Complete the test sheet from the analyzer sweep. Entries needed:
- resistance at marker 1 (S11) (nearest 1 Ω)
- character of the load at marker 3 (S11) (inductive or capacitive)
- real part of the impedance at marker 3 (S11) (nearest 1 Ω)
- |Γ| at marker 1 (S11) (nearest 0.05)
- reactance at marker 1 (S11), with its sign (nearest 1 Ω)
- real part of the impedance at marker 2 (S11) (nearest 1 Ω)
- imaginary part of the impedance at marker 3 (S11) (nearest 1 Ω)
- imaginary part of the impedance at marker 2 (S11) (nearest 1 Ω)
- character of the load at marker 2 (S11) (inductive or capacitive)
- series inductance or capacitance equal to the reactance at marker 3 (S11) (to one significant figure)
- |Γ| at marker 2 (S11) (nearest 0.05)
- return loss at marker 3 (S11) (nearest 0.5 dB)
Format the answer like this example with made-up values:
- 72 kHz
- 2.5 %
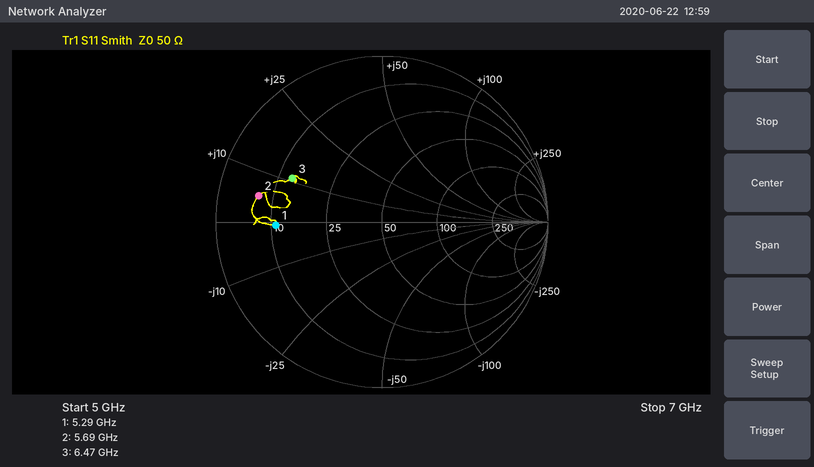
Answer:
- 11 Ω
- inductive
- 13 Ω
- 0.65
- -1 Ω
- 7 Ω
- +11 Ω
- +5 Ω
- inductive
- 300 pH
- 0.75
- 4.5 dB
